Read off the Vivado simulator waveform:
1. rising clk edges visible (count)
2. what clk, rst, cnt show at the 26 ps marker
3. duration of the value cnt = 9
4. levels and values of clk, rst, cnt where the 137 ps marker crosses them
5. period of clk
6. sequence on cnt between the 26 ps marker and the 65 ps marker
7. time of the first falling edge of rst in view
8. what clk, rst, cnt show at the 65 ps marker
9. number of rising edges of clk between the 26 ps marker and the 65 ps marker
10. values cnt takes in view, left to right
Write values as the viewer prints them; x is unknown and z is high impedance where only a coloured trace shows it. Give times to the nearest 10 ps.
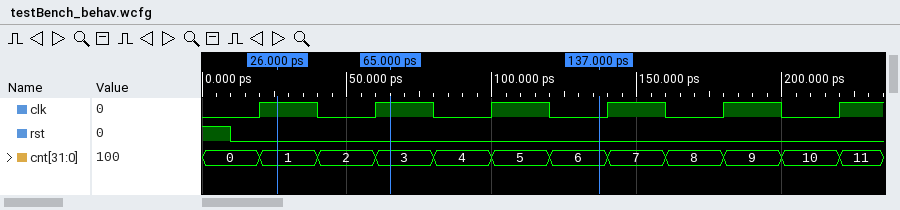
6
clk=1, rst=0, cnt=1
20 ps
clk=0, rst=0, cnt=6
40 ps
1, 2, 3
10 ps
clk=1, rst=0, cnt=3
1
0, 1, 2, 3, 4, 5, 6, 7, 8, 9, 10, 11
